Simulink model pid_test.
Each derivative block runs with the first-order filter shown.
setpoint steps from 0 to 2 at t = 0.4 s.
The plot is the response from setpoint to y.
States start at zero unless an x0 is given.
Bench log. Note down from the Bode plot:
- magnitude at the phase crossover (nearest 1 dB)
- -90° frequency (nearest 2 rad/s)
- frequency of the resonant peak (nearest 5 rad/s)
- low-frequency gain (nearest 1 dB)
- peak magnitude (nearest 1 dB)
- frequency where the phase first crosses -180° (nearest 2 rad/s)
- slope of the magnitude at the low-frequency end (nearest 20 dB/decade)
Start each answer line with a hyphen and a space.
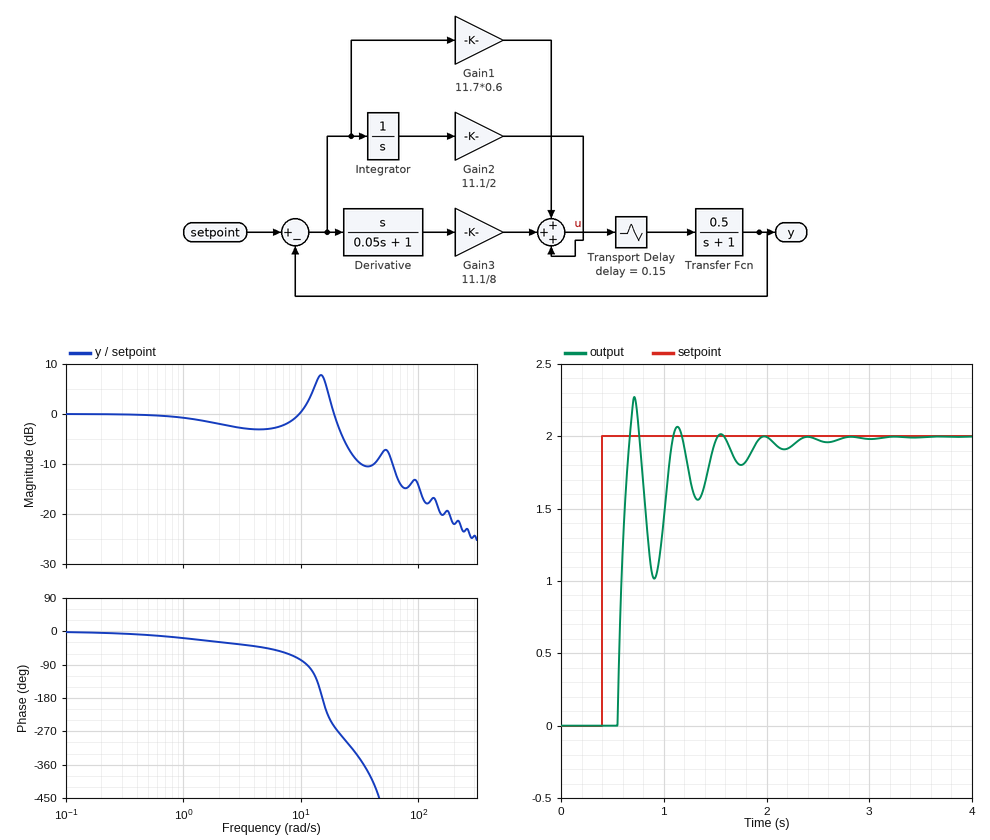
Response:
- 8 dB
- 12 rad/s
- 15 rad/s
- 0 dB
- 8 dB
- 16 rad/s
- 0 dB/decade
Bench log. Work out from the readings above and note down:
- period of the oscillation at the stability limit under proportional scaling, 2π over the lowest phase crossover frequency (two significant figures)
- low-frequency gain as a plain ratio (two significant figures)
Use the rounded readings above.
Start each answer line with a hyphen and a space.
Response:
- 0.39 s
- 1.0
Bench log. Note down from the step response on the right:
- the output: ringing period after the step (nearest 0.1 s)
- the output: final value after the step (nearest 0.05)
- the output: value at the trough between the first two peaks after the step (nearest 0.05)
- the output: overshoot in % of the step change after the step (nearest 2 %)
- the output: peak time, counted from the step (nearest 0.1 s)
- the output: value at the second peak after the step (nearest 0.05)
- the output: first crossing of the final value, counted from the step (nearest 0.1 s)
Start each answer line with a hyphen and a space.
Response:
- 0.4 s
- 2.00
- 1.00
- 14 %
- 0.3 s
- 2.05
- 0.3 s
